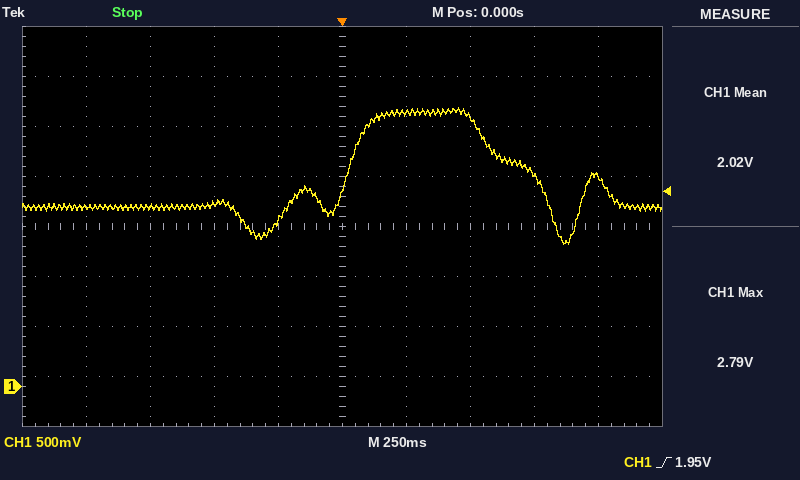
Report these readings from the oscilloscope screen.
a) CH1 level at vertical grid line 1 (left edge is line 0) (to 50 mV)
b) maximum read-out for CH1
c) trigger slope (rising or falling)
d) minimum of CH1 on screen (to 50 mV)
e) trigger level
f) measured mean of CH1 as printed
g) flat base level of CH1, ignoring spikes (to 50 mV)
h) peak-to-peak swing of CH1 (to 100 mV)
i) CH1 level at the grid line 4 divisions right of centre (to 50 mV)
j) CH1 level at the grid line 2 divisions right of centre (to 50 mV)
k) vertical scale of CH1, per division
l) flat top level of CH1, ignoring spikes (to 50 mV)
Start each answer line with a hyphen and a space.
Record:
- 1.80 V
- 2.79 V
- rising
- 1.40 V
- 1.95 V
- 2.02 V
- 1.80 V
- 1.40 V
- 2.10 V
- 2.70 V
- 500 mV
- 2.75 V
